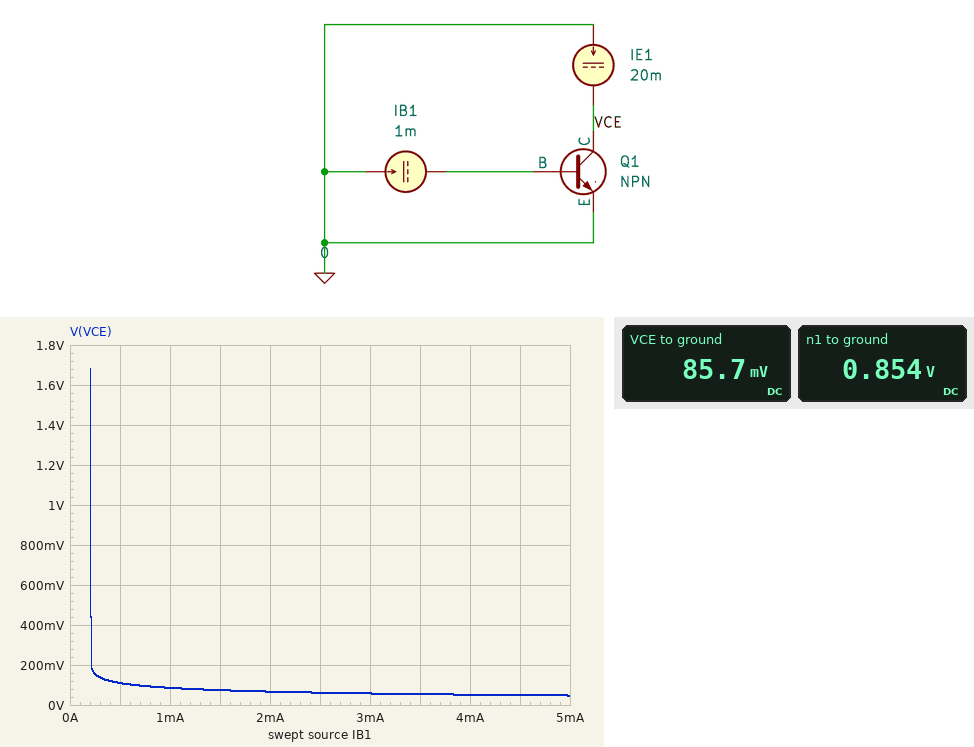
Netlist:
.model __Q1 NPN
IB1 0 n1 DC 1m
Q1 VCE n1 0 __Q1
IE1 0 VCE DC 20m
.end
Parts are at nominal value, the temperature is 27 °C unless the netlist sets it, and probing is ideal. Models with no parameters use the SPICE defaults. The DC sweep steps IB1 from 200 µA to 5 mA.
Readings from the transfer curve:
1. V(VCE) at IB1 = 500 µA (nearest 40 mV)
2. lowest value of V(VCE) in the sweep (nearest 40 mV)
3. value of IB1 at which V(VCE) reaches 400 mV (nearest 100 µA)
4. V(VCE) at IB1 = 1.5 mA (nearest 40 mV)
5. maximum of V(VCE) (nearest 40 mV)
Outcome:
120 mV
40 mV
200 µA
80 mV
1.68 V
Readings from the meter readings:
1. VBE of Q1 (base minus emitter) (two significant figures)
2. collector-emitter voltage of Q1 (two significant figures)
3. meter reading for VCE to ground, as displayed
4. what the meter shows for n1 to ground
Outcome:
850 mV
86 mV
85.7 mV
0.854 V
